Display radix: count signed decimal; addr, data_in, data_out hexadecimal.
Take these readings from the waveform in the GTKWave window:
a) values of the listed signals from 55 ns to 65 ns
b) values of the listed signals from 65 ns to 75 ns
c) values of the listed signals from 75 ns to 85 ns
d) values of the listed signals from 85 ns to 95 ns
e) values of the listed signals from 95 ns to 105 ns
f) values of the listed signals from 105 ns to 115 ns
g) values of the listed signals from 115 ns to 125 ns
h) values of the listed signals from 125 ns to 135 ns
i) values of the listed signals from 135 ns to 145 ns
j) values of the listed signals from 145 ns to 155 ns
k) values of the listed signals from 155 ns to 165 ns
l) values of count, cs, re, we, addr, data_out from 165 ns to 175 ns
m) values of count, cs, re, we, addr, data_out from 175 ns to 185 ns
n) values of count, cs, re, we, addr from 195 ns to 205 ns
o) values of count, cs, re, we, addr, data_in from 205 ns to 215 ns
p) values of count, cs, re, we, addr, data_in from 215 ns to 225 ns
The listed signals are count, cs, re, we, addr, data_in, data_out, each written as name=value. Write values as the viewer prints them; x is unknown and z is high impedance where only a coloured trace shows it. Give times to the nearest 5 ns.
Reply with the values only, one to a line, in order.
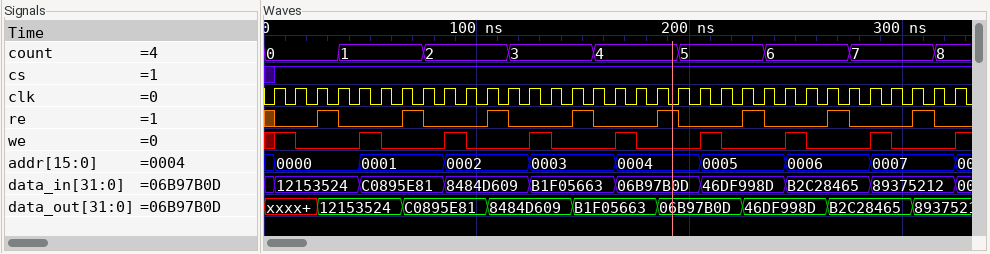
count=1, cs=1, re=0, we=0, addr=0001, data_in=C0895E81, data_out=12153524
count=1, cs=1, re=1, we=0, addr=0001, data_in=C0895E81, data_out=C0895E81
count=2, cs=1, re=0, we=0, addr=0001, data_in=C0895E81, data_out=C0895E81
count=2, cs=1, re=0, we=1, addr=0002, data_in=8484D609, data_out=C0895E81
count=2, cs=1, re=0, we=0, addr=0002, data_in=8484D609, data_out=C0895E81
count=2, cs=1, re=1, we=0, addr=0002, data_in=8484D609, data_out=8484D609
count=3, cs=1, re=0, we=0, addr=0002, data_in=8484D609, data_out=8484D609
count=3, cs=1, re=0, we=1, addr=0003, data_in=B1F05663, data_out=8484D609
count=3, cs=1, re=0, we=0, addr=0003, data_in=B1F05663, data_out=8484D609
count=3, cs=1, re=1, we=0, addr=0003, data_in=B1F05663, data_out=B1F05663
count=4, cs=1, re=0, we=0, addr=0003, data_in=B1F05663, data_out=B1F05663
count=4, cs=1, re=0, we=1, addr=0004, data_out=B1F05663
count=4, cs=1, re=0, we=0, addr=0004, data_out=B1F05663
count=5, cs=1, re=0, we=0, addr=0004
count=5, cs=1, re=0, we=1, addr=0005, data_in=46DF998D
count=5, cs=1, re=0, we=0, addr=0005, data_in=46DF998D
